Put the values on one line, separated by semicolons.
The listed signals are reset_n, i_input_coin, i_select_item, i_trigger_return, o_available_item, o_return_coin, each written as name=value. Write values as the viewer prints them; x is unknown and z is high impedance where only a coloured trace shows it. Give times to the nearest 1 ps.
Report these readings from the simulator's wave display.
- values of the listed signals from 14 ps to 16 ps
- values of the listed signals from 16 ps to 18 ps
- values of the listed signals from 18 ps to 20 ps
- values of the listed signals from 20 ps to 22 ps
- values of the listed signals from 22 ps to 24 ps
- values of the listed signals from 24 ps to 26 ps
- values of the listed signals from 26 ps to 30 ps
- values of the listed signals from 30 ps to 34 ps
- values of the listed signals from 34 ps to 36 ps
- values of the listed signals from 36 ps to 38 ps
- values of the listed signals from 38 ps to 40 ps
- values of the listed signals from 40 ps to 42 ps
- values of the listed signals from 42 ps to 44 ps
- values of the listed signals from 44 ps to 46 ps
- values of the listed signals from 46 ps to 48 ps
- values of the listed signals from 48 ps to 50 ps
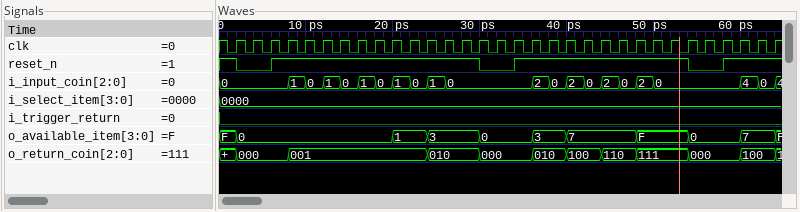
reset_n=1, i_input_coin=0, i_select_item=0000, i_trigger_return=0, o_available_item=0, o_return_coin=001; reset_n=1, i_input_coin=1, i_select_item=0000, i_trigger_return=0, o_available_item=0, o_return_coin=001; reset_n=1, i_input_coin=0, i_select_item=0000, i_trigger_return=0, o_available_item=0, o_return_coin=001; reset_n=1, i_input_coin=1, i_select_item=0000, i_trigger_return=0, o_available_item=1, o_return_coin=001; reset_n=1, i_input_coin=0, i_select_item=0000, i_trigger_return=0, o_available_item=1, o_return_coin=001; reset_n=1, i_input_coin=1, i_select_item=0000, i_trigger_return=0, o_available_item=3, o_return_coin=010; reset_n=1, i_input_coin=0, i_select_item=0000, i_trigger_return=0, o_available_item=3, o_return_coin=010; reset_n=0, i_input_coin=0, i_select_item=0000, i_trigger_return=0, o_available_item=0, o_return_coin=000; reset_n=1, i_input_coin=0, i_select_item=0000, i_trigger_return=0, o_available_item=0, o_return_coin=000; reset_n=1, i_input_coin=2, i_select_item=0000, i_trigger_return=0, o_available_item=3, o_return_coin=010; reset_n=1, i_input_coin=0, i_select_item=0000, i_trigger_return=0, o_available_item=3, o_return_coin=010; reset_n=1, i_input_coin=2, i_select_item=0000, i_trigger_return=0, o_available_item=7, o_return_coin=100; reset_n=1, i_input_coin=0, i_select_item=0000, i_trigger_return=0, o_available_item=7, o_return_coin=100; reset_n=1, i_input_coin=2, i_select_item=0000, i_trigger_return=0, o_available_item=7, o_return_coin=110; reset_n=1, i_input_coin=0, i_select_item=0000, i_trigger_return=0, o_available_item=7, o_return_coin=110; reset_n=1, i_input_coin=2, i_select_item=0000, i_trigger_return=0, o_available_item=F, o_return_coin=111
